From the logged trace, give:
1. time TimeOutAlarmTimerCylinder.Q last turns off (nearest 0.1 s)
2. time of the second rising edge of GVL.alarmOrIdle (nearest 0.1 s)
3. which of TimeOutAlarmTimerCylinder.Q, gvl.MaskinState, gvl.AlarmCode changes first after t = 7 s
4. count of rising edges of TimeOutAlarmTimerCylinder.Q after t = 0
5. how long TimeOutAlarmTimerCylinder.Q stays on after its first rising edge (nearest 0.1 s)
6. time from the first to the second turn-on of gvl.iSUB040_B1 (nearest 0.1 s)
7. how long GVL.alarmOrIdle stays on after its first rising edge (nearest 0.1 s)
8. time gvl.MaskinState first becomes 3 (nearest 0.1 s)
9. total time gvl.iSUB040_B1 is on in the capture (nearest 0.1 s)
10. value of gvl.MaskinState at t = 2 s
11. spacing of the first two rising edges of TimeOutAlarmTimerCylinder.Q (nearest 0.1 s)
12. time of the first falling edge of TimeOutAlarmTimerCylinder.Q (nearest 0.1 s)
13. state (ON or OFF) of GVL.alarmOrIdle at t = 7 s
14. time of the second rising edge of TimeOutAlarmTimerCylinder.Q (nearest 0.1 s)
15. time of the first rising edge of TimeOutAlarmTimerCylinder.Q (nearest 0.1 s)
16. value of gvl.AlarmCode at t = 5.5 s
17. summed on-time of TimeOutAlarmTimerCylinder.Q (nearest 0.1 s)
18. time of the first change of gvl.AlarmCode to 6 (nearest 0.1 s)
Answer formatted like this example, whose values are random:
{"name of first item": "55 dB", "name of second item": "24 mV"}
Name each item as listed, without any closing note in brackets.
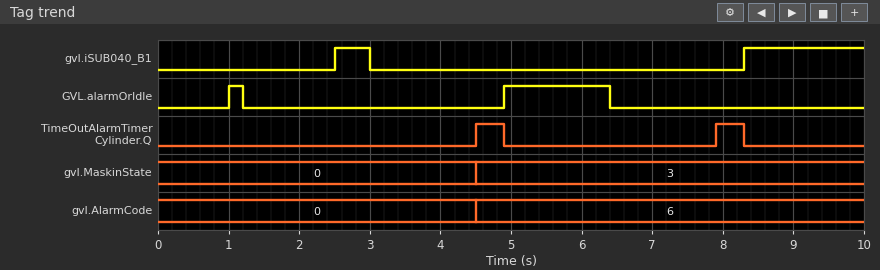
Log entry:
{"time TimeOutAlarmTimerCylinder.Q last turns off": "8.3 s", "time of the second rising edge of GVL.alarmOrIdle": "4.9 s", "which of TimeOutAlarmTimerCylinder.Q, gvl.MaskinState, gvl.AlarmCode changes first after t = 7 s": "TimeOutAlarmTimerCylinder.Q", "count of rising edges of TimeOutAlarmTimerCylinder.Q after t = 0": "2", "how long TimeOutAlarmTimerCylinder.Q stays on after its first rising edge": "0.4 s", "time from the first to the second turn-on of gvl.iSUB040_B1": "5.8 s", "how long GVL.alarmOrIdle stays on after its first rising edge": "0.2 s", "time gvl.MaskinState first becomes 3": "4.5 s", "total time gvl.iSUB040_B1 is on in the capture": "2.2 s", "value of gvl.MaskinState at t = 2 s": "0", "spacing of the first two rising edges of TimeOutAlarmTimerCylinder.Q": "3.4 s", "time of the first falling edge of TimeOutAlarmTimerCylinder.Q": "4.9 s", "state (ON or OFF) of GVL.alarmOrIdle at t = 7 s": "OFF", "time of the second rising edge of TimeOutAlarmTimerCylinder.Q": "7.9 s", "time of the first rising edge of TimeOutAlarmTimerCylinder.Q": "4.5 s", "value of gvl.AlarmCode at t = 5.5 s": "6", "summed on-time of TimeOutAlarmTimerCylinder.Q": "0.8 s", "time of the first change of gvl.AlarmCode to 6": "4.5 s"}
